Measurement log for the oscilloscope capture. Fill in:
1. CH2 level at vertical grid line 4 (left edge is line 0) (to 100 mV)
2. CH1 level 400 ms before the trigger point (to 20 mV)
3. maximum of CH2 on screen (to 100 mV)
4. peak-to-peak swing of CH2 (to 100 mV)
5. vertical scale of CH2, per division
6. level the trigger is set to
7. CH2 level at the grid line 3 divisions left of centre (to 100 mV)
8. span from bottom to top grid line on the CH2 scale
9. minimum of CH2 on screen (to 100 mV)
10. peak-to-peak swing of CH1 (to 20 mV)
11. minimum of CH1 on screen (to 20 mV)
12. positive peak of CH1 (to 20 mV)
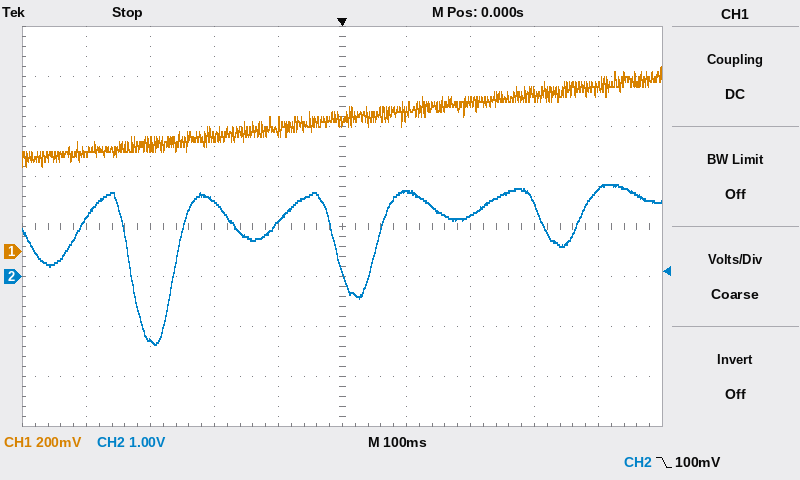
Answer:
1.1 V
400 mV
1.8 V
3.2 V
1 V
100 mV
-1.3 V
8 V
-1.4 V
400 mV
340 mV
740 mV
